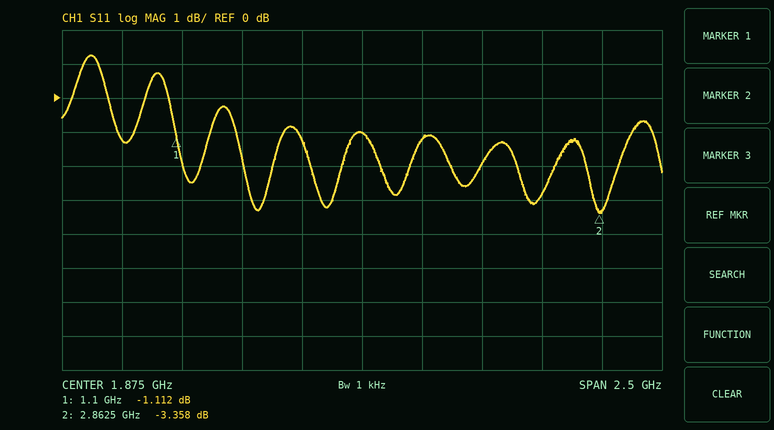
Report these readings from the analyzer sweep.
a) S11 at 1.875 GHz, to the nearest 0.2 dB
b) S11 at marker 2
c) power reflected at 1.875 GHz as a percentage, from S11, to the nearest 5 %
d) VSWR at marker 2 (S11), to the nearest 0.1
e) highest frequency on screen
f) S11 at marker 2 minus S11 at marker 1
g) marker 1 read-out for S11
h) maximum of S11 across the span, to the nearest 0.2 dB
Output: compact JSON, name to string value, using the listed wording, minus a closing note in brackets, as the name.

{"S11 at 1.875 GHz, to the nearest 0.2 dB": "-1.0 dB", "S11 at marker 2": "-3.358 dB", "power reflected at 1.875 GHz as a percentage, from S11, to the nearest 5 %": "80 %", "VSWR at marker 2 (S11), to the nearest 0.1": "5.2", "highest frequency on screen": "3.125 GHz", "S11 at marker 2 minus S11 at marker 1": "-2.246 dB", "marker 1 read-out for S11": "-1.112 dB", "maximum of S11 across the span, to the nearest 0.2 dB": "1.2 dB"}
